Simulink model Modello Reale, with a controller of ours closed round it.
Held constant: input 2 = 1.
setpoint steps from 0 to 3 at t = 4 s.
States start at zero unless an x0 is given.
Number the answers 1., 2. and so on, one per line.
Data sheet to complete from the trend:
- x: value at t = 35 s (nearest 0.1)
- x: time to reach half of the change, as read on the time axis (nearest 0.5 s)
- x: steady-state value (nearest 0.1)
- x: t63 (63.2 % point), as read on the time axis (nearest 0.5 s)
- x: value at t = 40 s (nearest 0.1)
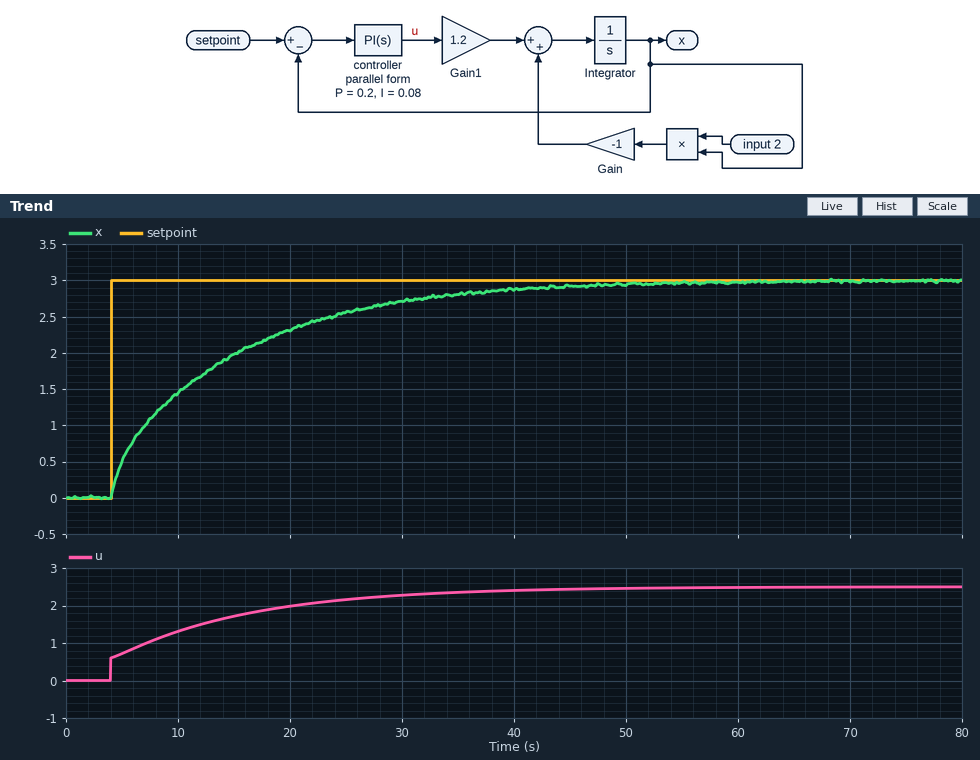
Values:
1. 2.8
2. 10.5 s
3. 3.0
4. 14.0 s
5. 2.9
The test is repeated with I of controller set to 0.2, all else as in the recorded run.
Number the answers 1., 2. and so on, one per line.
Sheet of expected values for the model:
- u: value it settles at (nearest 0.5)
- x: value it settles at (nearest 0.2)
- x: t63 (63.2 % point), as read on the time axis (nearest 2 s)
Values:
1. 2.5
2. 3.0
3. 8 s
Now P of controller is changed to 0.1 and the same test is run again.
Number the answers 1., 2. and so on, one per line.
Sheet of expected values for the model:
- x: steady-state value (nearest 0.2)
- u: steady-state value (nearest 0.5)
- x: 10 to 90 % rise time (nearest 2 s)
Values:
1. 3.0
2. 2.5
3. 24 s
